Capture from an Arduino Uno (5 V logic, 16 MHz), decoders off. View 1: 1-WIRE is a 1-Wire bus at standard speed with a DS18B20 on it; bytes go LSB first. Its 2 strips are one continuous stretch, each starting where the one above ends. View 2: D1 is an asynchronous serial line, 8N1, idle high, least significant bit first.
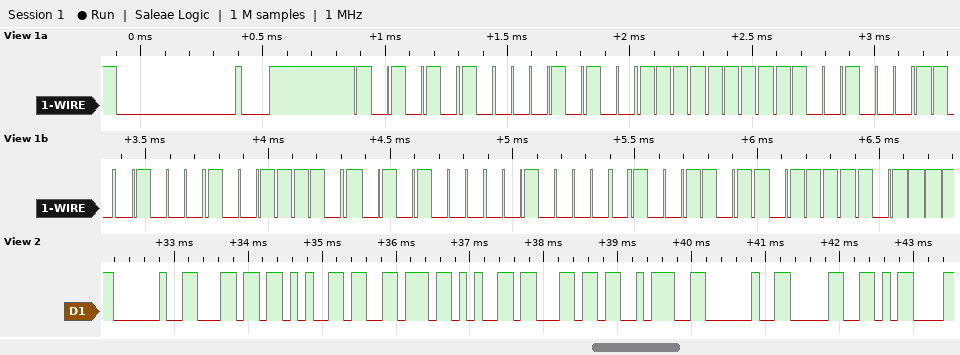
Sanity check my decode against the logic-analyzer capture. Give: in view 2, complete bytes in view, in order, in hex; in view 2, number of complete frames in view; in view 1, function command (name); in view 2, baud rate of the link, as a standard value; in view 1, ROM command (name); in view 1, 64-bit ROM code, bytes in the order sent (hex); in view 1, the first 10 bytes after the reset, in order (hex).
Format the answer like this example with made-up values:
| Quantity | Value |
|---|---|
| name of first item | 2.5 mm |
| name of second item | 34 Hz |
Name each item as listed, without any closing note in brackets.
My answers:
| Quantity | Value |
|---|---|
| in view 2, complete bytes in view, in order, in hex | 20 6C 65 76 65 6C 3A 20 30 0D |
| in view 2, number of complete frames in view | 10 |
| in view 1, function command | Read Scratchpad |
| in view 2, baud rate of the link, as a standard value | 9600 baud |
| in view 1, ROM command | Match ROM |
| in view 1, 64-bit ROM code, bytes in the order sent | 28 FF 13 13 79 15 04 D9 |
| in view 1, the first 10 bytes after the reset, in order | 55 28 FF 13 13 79 15 04 D9 BE |
